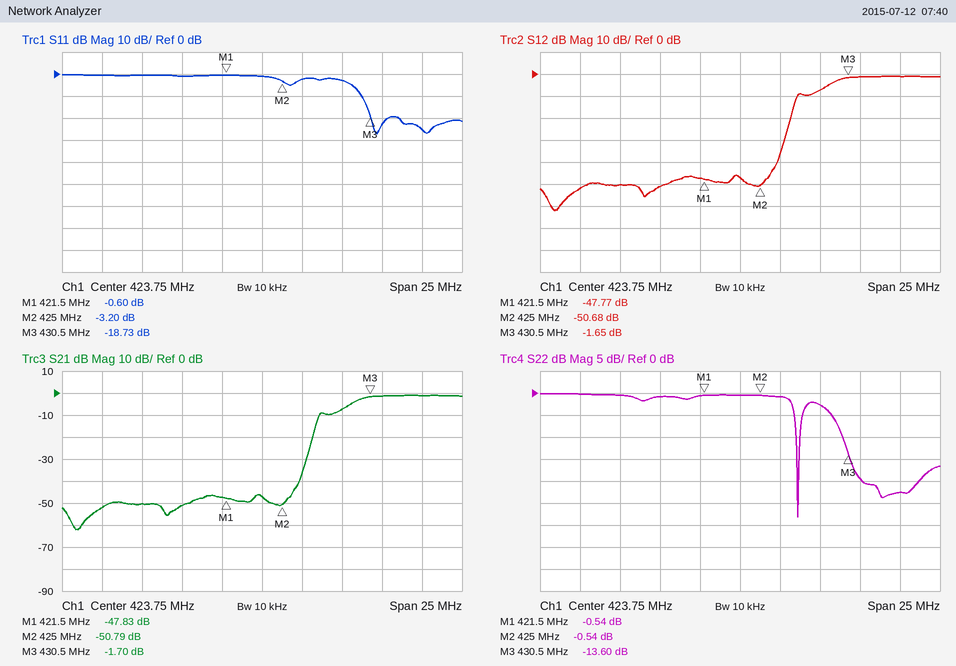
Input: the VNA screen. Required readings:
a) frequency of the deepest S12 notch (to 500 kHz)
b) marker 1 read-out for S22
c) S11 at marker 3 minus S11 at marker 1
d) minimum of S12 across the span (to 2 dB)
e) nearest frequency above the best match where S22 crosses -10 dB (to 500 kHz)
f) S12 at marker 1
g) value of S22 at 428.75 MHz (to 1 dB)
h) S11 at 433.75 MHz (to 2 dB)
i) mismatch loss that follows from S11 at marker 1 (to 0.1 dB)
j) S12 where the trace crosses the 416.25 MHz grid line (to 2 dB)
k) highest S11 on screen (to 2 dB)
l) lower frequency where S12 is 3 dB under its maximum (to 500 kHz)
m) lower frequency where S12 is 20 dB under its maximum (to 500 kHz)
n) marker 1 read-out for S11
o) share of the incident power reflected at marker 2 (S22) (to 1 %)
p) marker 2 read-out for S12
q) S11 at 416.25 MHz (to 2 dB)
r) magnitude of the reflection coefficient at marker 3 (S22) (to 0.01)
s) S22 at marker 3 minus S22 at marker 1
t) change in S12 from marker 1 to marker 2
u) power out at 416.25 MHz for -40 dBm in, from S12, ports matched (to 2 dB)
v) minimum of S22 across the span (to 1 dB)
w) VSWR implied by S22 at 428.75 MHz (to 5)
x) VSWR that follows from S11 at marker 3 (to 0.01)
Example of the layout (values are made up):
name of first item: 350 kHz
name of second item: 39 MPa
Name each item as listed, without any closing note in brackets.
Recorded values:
frequency of the deepest S12 notch: 412.0 MHz
marker 1 read-out for S22: -0.54 dB
S11 at marker 3 minus S11 at marker 1: -18.13 dB
minimum of S12 across the span: -62 dB
nearest frequency above the best match where S22 crosses -10 dB: 427.5 MHz
S12 at marker 1: -47.77 dB
value of S22 at 428.75 MHz: -3 dB
S11 at 433.75 MHz: -26 dB
mismatch loss that follows from S11 at marker 1: 8.9 dB
S12 where the trace crosses the 416.25 MHz grid line: -50 dB
highest S11 on screen: 0 dB
lower frequency where S12 is 3 dB under its maximum: 429.5 MHz
lower frequency where S12 is 20 dB under its maximum: 427.0 MHz
marker 1 read-out for S11: -0.60 dB
share of the incident power reflected at marker 2 (S22): 88 %
marker 2 read-out for S12: -50.68 dB
S11 at 416.25 MHz: 0 dB
magnitude of the reflection coefficient at marker 3 (S22): 0.21
S22 at marker 3 minus S22 at marker 1: -13.06 dB
change in S12 from marker 1 to marker 2: -2.91 dB
power out at 416.25 MHz for -40 dBm in, from S12, ports matched: -90 dBm
minimum of S22 across the span: -28 dB
VSWR implied by S22 at 428.75 MHz: 5
VSWR that follows from S11 at marker 3: 1.26
